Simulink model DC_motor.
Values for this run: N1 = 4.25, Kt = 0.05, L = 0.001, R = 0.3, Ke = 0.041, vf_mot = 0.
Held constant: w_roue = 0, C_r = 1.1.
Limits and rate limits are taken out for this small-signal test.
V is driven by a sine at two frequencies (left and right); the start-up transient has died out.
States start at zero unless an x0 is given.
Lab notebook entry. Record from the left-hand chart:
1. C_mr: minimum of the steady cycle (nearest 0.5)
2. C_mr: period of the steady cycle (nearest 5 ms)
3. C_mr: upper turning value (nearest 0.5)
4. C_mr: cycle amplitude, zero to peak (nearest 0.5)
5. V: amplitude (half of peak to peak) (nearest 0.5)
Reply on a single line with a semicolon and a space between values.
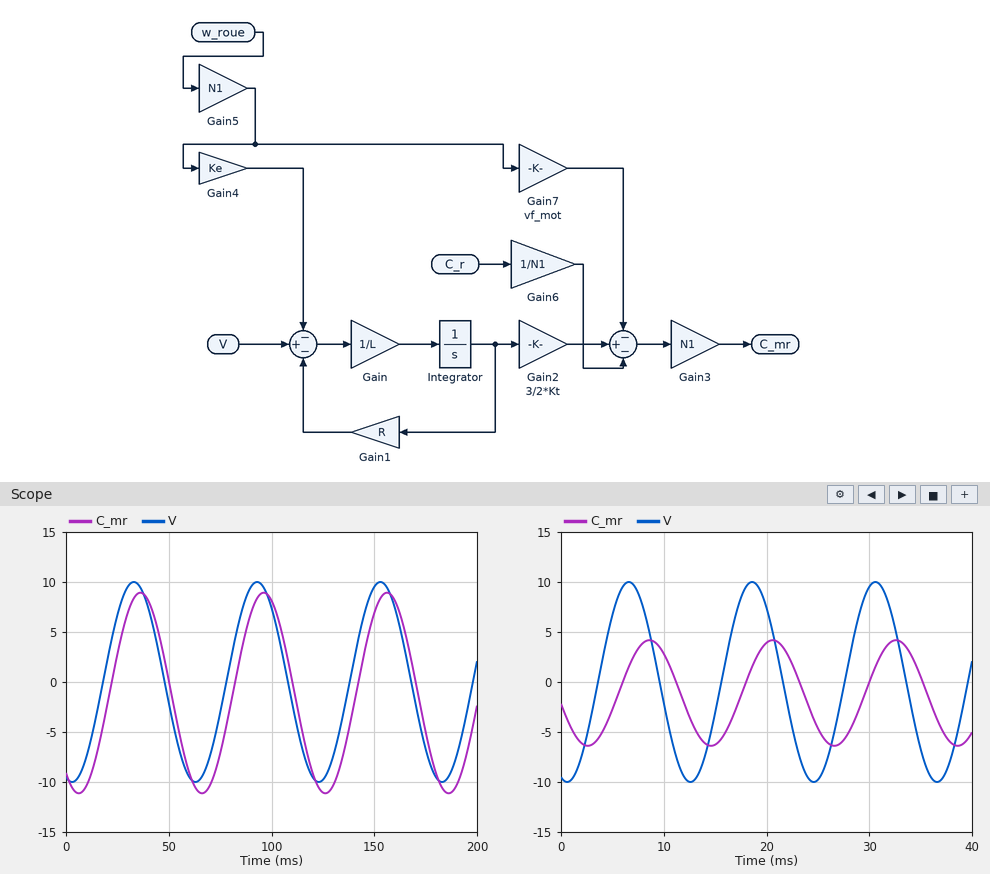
-11.0; 60 ms; 9.0; 10.0; 10.0
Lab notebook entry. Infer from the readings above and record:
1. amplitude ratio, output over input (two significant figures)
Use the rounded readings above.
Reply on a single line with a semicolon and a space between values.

1.0
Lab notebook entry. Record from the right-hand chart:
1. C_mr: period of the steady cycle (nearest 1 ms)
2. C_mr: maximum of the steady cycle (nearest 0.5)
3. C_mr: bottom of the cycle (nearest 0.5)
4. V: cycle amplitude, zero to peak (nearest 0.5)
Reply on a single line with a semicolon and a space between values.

12 ms; 4.0; -6.5; 10.0
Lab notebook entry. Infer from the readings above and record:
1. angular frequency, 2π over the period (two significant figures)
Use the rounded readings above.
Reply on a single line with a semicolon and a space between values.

0.52 rad/ms
